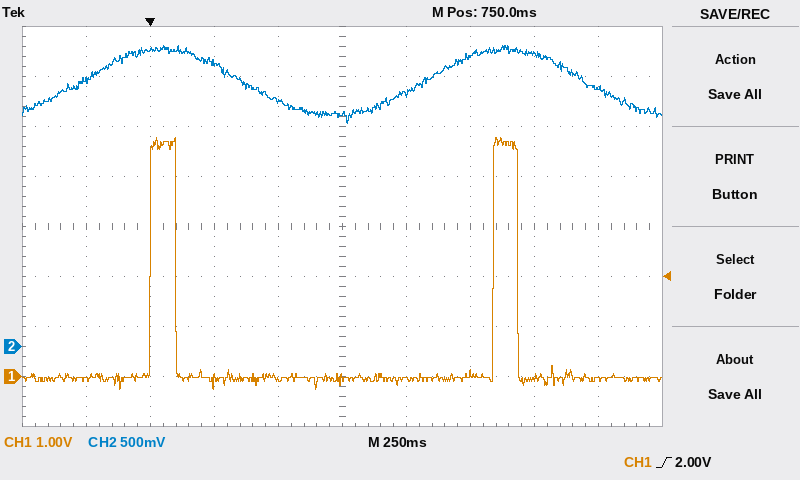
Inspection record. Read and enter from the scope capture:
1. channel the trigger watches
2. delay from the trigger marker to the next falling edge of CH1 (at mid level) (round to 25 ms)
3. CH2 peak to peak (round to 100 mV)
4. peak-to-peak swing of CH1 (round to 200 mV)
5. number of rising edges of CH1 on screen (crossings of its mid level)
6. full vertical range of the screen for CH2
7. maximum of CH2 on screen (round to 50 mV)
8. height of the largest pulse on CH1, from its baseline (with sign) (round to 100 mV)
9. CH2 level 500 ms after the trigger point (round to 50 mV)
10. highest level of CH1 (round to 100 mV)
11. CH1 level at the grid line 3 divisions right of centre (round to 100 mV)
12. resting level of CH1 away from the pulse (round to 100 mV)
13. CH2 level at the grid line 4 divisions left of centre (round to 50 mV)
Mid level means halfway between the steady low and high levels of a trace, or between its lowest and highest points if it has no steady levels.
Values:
CH1
100 ms
800 mV
5.0 V
2
4 V
3.00 V
+4.8 V
2.45 V
4.8 V
0.0 V
0.0 V
2.65 V
